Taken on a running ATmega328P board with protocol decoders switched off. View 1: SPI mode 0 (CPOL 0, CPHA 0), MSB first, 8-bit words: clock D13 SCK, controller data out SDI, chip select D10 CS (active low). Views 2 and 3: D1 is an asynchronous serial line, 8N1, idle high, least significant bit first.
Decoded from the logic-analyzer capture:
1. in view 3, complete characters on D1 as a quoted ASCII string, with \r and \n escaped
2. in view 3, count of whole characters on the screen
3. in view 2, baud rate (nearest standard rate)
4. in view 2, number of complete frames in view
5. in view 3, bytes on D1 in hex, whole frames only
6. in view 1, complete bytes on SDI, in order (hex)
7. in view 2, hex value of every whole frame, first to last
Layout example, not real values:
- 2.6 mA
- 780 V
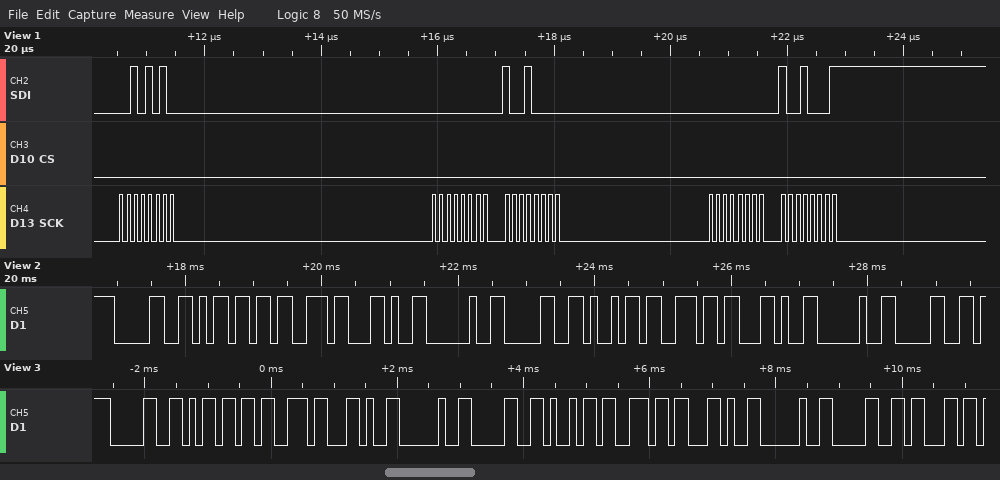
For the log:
- "0ms, 0in, 0c"
- 12
- 9600 baud
- 11
- 0x30 0x6D 0x73 0x2C 0x20 0x30 0x69 0x6E 0x2C 0x20 0x30 0x63
- 2A 00 90 00 91
- 0x30 0x6D 0x73 0x2C 0x20 0x30 0x69 0x6E 0x2C 0x20 0x30
